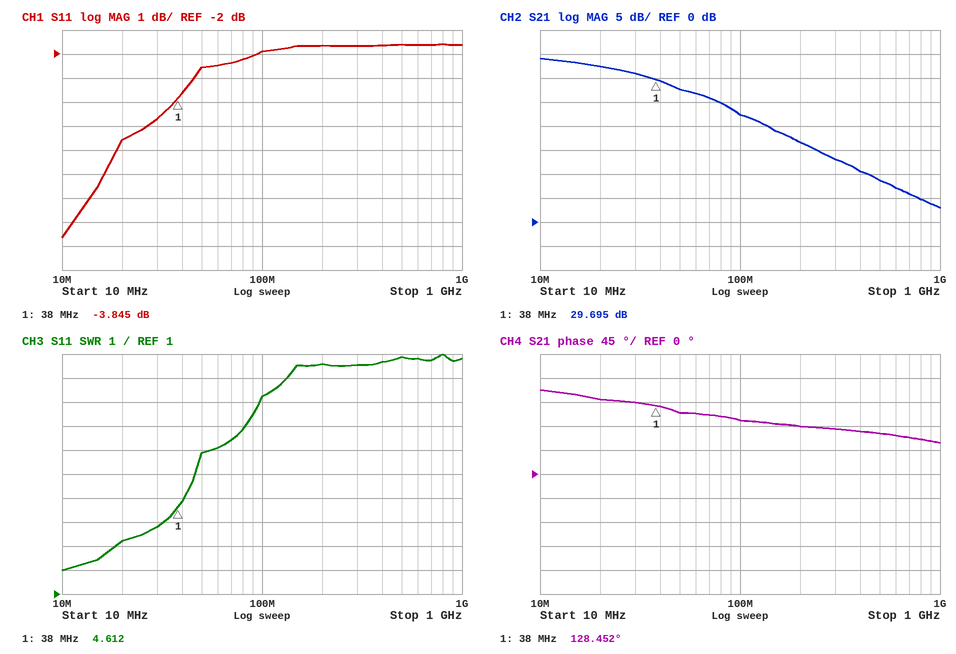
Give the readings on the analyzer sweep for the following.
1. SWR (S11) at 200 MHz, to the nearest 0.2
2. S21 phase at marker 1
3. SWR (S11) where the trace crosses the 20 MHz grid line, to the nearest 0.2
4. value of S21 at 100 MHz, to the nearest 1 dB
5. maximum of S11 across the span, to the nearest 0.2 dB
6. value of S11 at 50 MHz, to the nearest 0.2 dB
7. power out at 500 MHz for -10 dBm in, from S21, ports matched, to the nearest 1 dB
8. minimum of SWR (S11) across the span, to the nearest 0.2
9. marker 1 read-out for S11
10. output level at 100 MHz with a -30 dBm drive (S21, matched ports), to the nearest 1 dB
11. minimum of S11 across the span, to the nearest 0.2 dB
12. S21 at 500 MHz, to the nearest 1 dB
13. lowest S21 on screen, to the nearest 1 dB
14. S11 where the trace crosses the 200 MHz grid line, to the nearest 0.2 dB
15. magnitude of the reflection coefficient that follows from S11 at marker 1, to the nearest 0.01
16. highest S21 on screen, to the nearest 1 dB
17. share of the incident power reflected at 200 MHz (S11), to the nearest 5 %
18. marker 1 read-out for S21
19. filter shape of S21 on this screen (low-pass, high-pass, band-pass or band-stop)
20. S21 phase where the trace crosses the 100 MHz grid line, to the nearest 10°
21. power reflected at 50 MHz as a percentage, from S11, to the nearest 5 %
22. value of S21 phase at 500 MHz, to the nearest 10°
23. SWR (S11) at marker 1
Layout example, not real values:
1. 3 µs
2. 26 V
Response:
1. 10.6
2. 128.452°
3. 3.2
4. 22 dB
5. -1.6 dB
6. -2.6 dB
7. -1 dBm
8. 2.0
9. -3.845 dB
10. -8 dBm
11. -9.6 dB
12. 9 dB
13. 3 dB
14. -1.6 dB
15. 0.64
16. 34 dB
17. 70 %
18. 29.695 dB
19. low-pass
20. 100°
21. 55 %
22. 80°
23. 4.612
